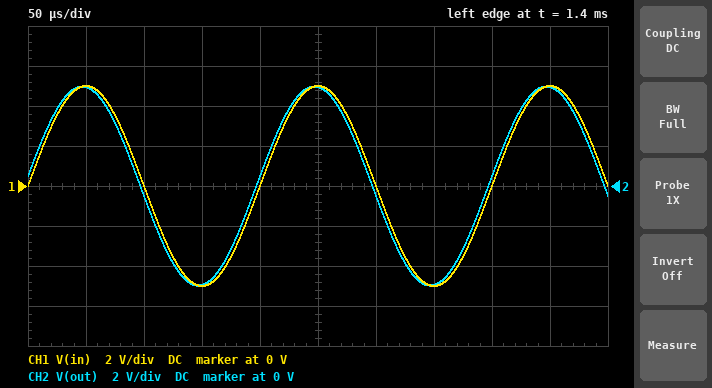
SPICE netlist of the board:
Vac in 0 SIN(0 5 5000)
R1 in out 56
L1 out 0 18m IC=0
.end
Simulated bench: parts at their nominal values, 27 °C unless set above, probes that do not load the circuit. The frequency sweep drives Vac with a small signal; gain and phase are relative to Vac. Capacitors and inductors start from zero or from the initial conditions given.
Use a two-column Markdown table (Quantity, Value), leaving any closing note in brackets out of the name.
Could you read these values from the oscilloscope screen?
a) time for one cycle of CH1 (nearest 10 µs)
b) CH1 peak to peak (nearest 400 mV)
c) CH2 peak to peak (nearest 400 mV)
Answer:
| Quantity | Value |
|---|---|
| time for one cycle of CH1 | 200 µs |
| CH1 peak to peak | 10.0 V |
| CH2 peak to peak | 10.0 V |
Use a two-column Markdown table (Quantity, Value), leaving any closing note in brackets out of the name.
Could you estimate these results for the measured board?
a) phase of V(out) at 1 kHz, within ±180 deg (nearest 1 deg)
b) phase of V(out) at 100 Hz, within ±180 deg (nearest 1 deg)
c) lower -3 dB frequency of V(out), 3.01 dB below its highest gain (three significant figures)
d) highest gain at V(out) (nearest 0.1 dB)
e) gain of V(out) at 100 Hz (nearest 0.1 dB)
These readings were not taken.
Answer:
| Quantity | Value |
|---|---|
| phase of V(out) at 1 kHz, within ±180 deg | 26 deg |
| phase of V(out) at 100 Hz, within ±180 deg | 79 deg |
| lower -3 dB frequency of V(out), 3.01 dB below its highest gain | 495 Hz |
| highest gain at V(out) | 0 dB |
| gain of V(out) at 100 Hz | -14.1 dB |
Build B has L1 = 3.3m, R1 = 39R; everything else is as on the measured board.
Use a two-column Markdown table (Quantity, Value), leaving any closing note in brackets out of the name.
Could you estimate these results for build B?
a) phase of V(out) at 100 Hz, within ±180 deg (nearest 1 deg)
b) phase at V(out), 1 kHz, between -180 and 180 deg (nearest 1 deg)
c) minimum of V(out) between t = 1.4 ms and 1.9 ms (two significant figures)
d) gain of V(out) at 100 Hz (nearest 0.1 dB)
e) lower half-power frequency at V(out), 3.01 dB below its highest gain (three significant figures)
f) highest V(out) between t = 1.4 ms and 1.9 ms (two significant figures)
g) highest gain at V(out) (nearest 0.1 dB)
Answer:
| Quantity | Value |
|---|---|
| phase of V(out) at 100 Hz, within ±180 deg | 87 deg |
| phase at V(out), 1 kHz, between -180 and 180 deg | 62 deg |
| minimum of V(out) between t = 1.4 ms and 1.9 ms | -4.7 V |
| gain of V(out) at 100 Hz | -25.5 dB |
| lower half-power frequency at V(out), 3.01 dB below its highest gain | 1.88 kHz |
| highest V(out) between t = 1.4 ms and 1.9 ms | 4.7 V |
| highest gain at V(out) | 0 dB |
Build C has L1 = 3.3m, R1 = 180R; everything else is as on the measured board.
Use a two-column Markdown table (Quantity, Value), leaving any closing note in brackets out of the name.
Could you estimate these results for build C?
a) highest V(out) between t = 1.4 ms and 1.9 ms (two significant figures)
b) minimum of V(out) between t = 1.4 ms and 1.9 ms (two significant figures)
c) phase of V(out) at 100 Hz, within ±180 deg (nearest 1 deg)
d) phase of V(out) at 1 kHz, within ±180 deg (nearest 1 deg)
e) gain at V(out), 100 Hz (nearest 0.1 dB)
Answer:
| Quantity | Value |
|---|---|
| highest V(out) between t = 1.4 ms and 1.9 ms | 2.5 V |
| minimum of V(out) between t = 1.4 ms and 1.9 ms | -2.5 V |
| phase of V(out) at 100 Hz, within ±180 deg | 89 deg |
| phase of V(out) at 1 kHz, within ±180 deg | 83 deg |
| gain at V(out), 100 Hz | -38.8 dB |
